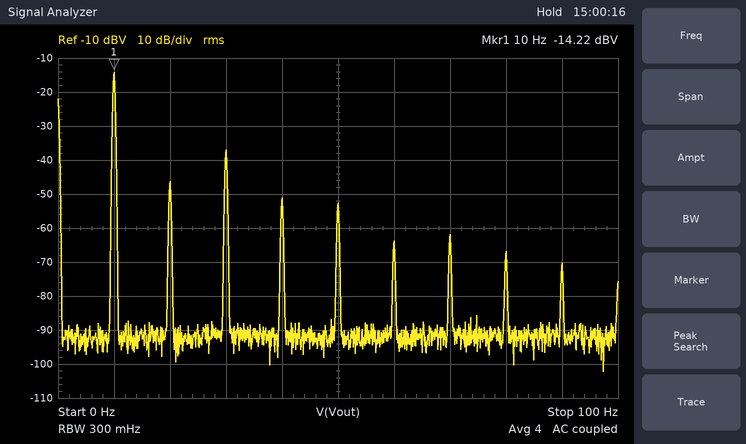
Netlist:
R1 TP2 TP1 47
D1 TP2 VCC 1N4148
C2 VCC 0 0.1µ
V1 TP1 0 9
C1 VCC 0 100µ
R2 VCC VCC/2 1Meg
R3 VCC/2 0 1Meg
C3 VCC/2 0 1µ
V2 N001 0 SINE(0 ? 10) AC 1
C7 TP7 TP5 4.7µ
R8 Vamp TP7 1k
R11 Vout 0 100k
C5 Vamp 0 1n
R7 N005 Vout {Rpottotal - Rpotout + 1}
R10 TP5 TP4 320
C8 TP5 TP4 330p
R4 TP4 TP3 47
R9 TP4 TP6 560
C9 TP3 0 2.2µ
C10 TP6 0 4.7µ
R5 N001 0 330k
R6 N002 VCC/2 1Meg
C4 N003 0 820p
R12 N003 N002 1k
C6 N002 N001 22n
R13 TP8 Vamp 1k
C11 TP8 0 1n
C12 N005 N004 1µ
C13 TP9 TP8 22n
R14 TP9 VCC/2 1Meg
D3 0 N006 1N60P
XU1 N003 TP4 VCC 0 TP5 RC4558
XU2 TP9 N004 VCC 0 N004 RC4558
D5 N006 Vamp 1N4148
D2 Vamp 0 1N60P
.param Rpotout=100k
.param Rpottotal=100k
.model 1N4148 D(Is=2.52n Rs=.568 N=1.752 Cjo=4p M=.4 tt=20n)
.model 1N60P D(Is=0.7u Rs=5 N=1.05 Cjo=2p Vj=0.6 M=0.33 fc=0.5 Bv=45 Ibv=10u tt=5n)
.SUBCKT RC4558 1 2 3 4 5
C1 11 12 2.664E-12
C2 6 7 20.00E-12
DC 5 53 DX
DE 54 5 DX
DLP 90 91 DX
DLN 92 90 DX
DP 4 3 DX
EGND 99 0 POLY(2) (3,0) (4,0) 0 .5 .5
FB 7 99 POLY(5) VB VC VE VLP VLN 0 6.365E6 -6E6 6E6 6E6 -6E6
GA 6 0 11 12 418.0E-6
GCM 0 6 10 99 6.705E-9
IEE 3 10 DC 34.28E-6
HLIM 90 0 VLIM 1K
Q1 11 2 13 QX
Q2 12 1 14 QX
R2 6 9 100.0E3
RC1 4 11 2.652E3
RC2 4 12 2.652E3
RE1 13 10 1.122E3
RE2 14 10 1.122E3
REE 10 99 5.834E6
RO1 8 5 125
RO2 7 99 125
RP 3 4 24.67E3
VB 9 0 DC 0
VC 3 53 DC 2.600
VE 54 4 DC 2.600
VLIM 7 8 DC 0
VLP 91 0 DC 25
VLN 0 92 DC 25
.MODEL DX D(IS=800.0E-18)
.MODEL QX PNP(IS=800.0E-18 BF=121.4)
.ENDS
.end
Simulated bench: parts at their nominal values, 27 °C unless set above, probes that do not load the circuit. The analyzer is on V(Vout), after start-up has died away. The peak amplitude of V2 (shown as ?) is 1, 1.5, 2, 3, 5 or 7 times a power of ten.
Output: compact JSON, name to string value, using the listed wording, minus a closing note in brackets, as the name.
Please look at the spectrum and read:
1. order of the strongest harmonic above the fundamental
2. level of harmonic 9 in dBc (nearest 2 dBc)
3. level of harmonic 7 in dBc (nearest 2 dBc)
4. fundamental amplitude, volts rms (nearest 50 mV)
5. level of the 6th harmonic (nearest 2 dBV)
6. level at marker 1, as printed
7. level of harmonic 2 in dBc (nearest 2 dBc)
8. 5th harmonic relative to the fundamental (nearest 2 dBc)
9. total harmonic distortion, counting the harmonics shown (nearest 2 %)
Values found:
{"order of the strongest harmonic above the fundamental": "3", "level of harmonic 9 in dBc": "-56 dBc", "level of harmonic 7 in dBc": "-48 dBc", "fundamental amplitude, volts rms": "200 mV", "level of the 6th harmonic": "-64 dBV", "level at marker 1, as printed": "-14.22 dBV", "level of harmonic 2 in dBc": "-32 dBc", "5th harmonic relative to the fundamental": "-38 dBc", "total harmonic distortion, counting the harmonics shown": "8 %"}
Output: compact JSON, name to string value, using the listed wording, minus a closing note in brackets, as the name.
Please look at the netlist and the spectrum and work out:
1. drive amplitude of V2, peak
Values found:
{"drive amplitude of V2, peak": "500 mV"}
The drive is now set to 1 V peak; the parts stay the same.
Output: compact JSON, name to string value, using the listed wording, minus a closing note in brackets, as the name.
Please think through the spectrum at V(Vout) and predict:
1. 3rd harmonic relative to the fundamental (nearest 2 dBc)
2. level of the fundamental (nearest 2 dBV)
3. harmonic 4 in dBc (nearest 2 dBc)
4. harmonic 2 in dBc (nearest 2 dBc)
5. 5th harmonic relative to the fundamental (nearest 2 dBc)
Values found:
{"3rd harmonic relative to the fundamental": "-14 dBc", "level of the fundamental": "-12 dBV", "harmonic 4 in dBc": "-40 dBc", "harmonic 2 in dBc": "-28 dBc", "5th harmonic relative to the fundamental": "-28 dBc"}
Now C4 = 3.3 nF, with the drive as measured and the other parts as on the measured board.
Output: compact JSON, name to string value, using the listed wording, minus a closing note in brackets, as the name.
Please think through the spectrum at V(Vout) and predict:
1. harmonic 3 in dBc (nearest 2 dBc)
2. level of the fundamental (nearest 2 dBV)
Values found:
{"harmonic 3 in dBc": "-24 dBc", "level of the fundamental": "-14 dBV"}
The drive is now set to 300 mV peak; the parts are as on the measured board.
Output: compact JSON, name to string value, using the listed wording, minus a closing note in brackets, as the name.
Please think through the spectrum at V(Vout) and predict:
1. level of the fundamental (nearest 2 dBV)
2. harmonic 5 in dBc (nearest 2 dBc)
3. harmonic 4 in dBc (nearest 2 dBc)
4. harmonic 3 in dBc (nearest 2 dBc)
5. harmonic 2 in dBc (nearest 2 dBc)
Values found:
{"level of the fundamental": "-18 dBV", "harmonic 5 in dBc": "-48 dBc", "harmonic 4 in dBc": "-44 dBc", "harmonic 3 in dBc": "-36 dBc", "harmonic 2 in dBc": "-36 dBc"}
